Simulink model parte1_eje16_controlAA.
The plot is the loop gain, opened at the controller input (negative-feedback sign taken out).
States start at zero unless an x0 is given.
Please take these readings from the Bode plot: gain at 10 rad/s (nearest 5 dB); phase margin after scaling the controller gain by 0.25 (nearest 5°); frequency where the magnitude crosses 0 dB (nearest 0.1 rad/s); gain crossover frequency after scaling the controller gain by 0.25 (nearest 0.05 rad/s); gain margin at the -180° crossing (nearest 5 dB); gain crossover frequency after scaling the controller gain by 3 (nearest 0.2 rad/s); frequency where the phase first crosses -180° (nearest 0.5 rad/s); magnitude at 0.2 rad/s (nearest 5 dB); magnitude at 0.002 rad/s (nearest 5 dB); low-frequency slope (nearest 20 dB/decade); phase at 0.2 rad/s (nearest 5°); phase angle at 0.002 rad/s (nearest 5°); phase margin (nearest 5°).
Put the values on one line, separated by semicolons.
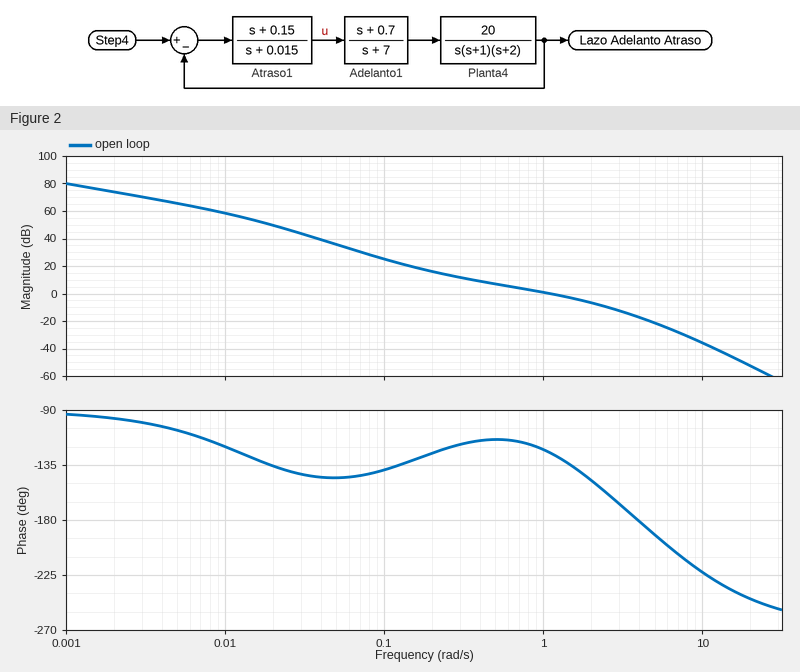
-35 dB; 60°; 1.1 rad/s; 0.30 rad/s; 15 dB; 2.4 rad/s; 4.0 rad/s; 15 dB; 75 dB; -20 dB/decade; -125°; -95°; 55°
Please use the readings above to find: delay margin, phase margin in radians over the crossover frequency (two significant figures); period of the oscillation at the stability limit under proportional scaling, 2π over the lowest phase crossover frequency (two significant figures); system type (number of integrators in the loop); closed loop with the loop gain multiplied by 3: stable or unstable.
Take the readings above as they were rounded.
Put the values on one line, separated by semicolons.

0.87 s; 1.6 s; 1; stable
